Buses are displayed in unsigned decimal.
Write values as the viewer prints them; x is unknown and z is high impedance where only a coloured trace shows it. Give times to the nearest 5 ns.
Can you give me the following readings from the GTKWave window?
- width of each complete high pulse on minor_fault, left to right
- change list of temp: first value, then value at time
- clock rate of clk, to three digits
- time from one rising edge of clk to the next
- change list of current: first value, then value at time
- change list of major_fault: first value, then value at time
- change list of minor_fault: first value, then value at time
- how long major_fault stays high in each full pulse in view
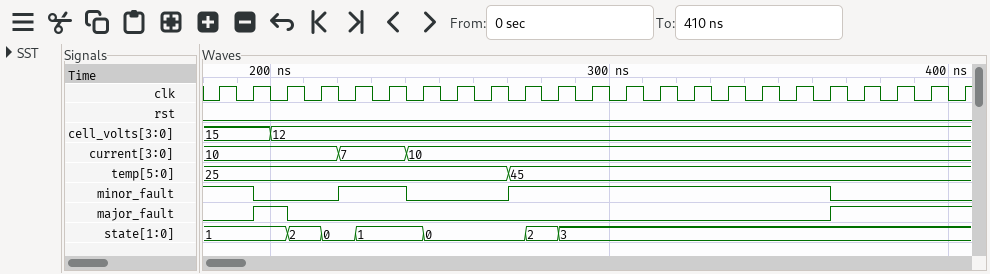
20 ns, 95 ns
25, 45 at 270 ns
100 MHz
10 ns
10, 7 at 220 ns, 10 at 240 ns
0, 1 at 195 ns, 0 at 205 ns, 1 at 365 ns
1, 0 at 195 ns, 1 at 220 ns, 0 at 240 ns, 1 at 270 ns, 0 at 365 ns
10 ns
